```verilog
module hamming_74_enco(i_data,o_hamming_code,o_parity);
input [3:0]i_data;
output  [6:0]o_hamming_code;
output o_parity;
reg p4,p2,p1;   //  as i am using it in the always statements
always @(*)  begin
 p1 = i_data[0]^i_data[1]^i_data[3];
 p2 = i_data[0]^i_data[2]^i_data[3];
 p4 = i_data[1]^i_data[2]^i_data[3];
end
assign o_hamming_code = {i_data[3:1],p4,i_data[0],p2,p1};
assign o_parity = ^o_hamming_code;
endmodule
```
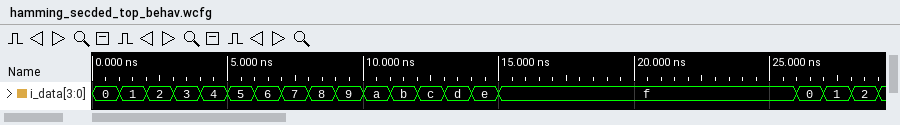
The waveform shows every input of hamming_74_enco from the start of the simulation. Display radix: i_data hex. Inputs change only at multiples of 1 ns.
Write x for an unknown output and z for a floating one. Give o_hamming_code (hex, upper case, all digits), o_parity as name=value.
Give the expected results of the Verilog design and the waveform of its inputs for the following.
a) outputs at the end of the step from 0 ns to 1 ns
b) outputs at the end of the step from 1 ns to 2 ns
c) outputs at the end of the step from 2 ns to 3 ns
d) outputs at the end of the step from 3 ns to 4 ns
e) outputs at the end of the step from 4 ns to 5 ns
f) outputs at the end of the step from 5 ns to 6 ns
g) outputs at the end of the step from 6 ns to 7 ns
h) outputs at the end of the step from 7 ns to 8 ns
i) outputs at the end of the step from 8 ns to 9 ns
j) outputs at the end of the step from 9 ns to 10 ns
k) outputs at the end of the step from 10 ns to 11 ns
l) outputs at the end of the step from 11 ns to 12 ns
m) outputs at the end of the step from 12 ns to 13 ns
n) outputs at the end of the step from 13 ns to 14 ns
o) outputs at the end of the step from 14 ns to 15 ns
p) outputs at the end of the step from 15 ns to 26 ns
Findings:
o_hamming_code=00, o_parity=0
o_hamming_code=07, o_parity=1
o_hamming_code=19, o_parity=1
o_hamming_code=1E, o_parity=0
o_hamming_code=2A, o_parity=1
o_hamming_code=2D, o_parity=0
o_hamming_code=33, o_parity=0
o_hamming_code=34, o_parity=1
o_hamming_code=4B, o_parity=0
o_hamming_code=4C, o_parity=1
o_hamming_code=52, o_parity=1
o_hamming_code=55, o_parity=0
o_hamming_code=61, o_parity=1
o_hamming_code=66, o_parity=0
o_hamming_code=78, o_parity=0
o_hamming_code=7F, o_parity=1
